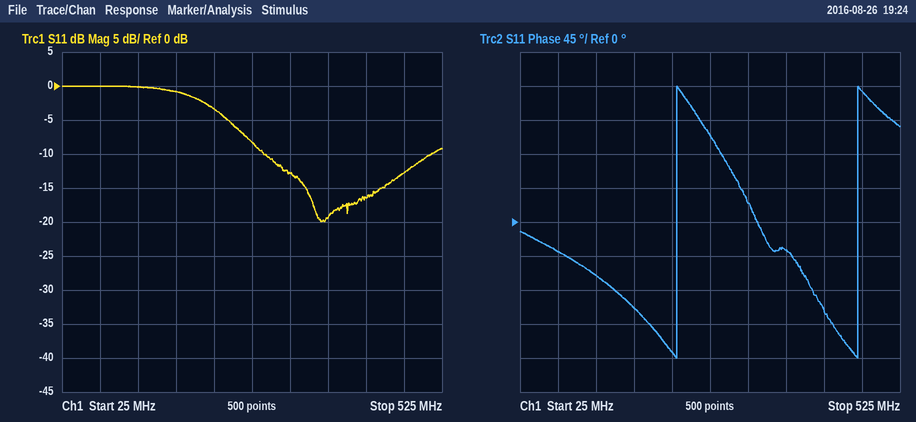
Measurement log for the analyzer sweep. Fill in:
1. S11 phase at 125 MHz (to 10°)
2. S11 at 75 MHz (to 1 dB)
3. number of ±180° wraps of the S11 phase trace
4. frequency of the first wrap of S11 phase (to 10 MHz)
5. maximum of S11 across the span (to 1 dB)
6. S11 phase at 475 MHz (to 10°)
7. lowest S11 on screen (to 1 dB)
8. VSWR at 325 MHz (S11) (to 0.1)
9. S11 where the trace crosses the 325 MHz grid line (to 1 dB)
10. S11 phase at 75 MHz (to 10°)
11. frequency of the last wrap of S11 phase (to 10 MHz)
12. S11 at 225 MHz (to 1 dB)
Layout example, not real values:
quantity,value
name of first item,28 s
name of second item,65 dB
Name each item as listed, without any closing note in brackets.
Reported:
quantity,value
S11 phase at 125 MHz,-70°
S11 at 75 MHz,0 dB
number of ±180° wraps of the S11 phase trace,2
frequency of the first wrap of S11 phase,230 MHz
maximum of S11 across the span,0 dB
S11 phase at 475 MHz,170°
lowest S11 on screen,-20 dB
VSWR at 325 MHz (S11),1.6
S11 where the trace crosses the 325 MHz grid line,-13 dB
S11 phase at 75 MHz,-40°
frequency of the last wrap of S11 phase,470 MHz
S11 at 225 MHz,-3 dB
